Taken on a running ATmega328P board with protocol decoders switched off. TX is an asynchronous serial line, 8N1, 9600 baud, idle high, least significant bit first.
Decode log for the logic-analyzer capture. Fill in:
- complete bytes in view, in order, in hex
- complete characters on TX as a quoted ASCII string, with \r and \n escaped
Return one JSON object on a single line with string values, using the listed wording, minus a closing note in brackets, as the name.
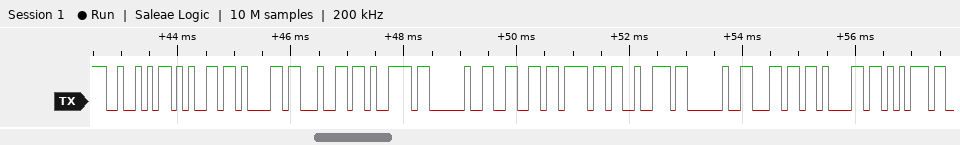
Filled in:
{"complete bytes in view, in order, in hex": "0x52 0x65 0x61 0x64 0x79 0x20 0x66 0x6F 0x72 0x20 0x6C 0x61 0x75", "complete characters on TX as a quoted ASCII string, with \\r and \\n escaped": "\"Ready for lau\""}
